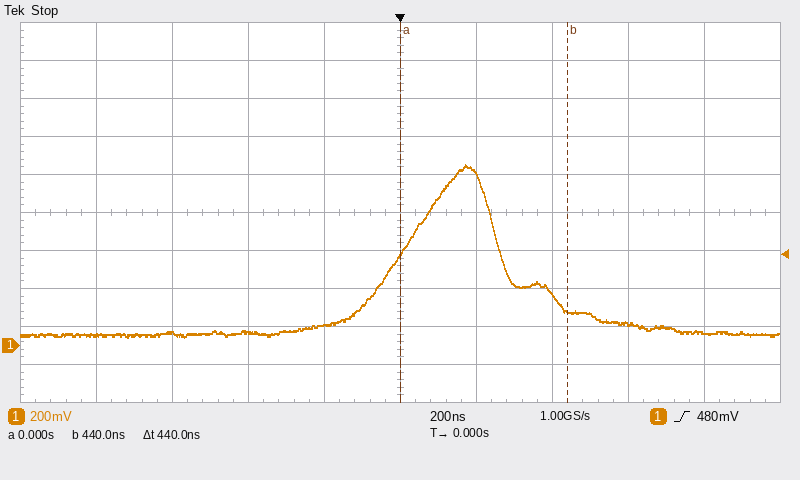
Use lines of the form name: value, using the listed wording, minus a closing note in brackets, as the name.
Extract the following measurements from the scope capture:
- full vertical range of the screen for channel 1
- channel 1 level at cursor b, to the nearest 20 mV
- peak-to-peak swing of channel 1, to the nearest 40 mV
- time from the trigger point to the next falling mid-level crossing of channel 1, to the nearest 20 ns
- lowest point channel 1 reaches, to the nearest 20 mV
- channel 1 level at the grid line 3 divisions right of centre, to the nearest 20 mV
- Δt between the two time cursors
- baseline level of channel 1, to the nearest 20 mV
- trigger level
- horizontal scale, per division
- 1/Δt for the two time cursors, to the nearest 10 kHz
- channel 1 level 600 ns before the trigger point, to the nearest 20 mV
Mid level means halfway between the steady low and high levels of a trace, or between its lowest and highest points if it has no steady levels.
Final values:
full vertical range of the screen for channel 1: 2 V
channel 1 level at cursor b, to the nearest 20 mV: 180 mV
peak-to-peak swing of channel 1, to the nearest 40 mV: 920 mV
time from the trigger point to the next falling mid-level crossing of channel 1, to the nearest 20 ns: 260 ns
lowest point channel 1 reaches, to the nearest 20 mV: 40 mV
channel 1 level at the grid line 3 divisions right of centre, to the nearest 20 mV: 120 mV
Δt between the two time cursors: 440 ns
baseline level of channel 1, to the nearest 20 mV: 60 mV
trigger level: 480 mV
horizontal scale, per division: 200 ns
1/Δt for the two time cursors, to the nearest 10 kHz: 2.27 MHz
channel 1 level 600 ns before the trigger point, to the nearest 20 mV: 60 mV
